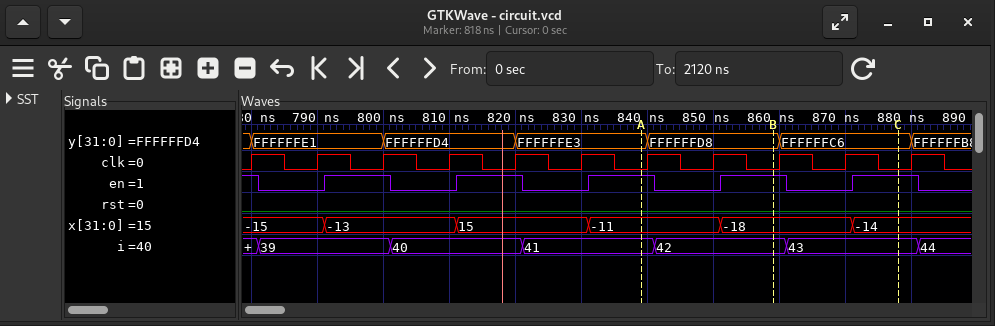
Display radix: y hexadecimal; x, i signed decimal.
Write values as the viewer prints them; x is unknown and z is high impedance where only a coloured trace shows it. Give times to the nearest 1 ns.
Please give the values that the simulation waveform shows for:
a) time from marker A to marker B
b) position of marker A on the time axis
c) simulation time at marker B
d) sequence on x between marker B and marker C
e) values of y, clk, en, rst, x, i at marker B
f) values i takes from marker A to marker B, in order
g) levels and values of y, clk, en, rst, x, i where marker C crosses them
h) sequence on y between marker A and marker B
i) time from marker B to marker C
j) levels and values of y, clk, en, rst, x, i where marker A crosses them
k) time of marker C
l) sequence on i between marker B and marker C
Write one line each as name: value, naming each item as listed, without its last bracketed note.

time from marker A to marker B: 20 ns
position of marker A on the time axis: 839 ns
simulation time at marker B: 859 ns
sequence on x between marker B and marker C: -18, -14
values of y, clk, en, rst, x, i at marker B: y=FFFFFFD8, clk=0, en=1, rst=0, x=-18, i=42
values i takes from marker A to marker B, in order: 41, 42
levels and values of y, clk, en, rst, x, i where marker C crosses them: y=FFFFFFC6, clk=0, en=1, rst=0, x=-14, i=43
sequence on y between marker A and marker B: FFFFFFE3, FFFFFFD8
time from marker B to marker C: 19 ns
levels and values of y, clk, en, rst, x, i where marker A crosses them: y=FFFFFFE3, clk=0, en=1, rst=0, x=-11, i=41
time of marker C: 878 ns
sequence on i between marker B and marker C: 42, 43
